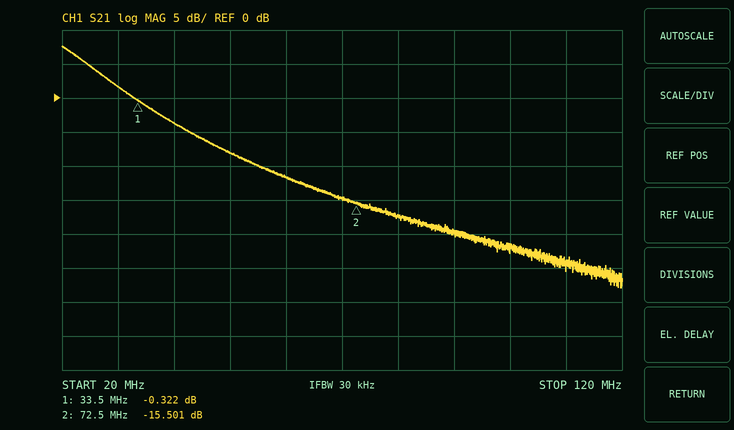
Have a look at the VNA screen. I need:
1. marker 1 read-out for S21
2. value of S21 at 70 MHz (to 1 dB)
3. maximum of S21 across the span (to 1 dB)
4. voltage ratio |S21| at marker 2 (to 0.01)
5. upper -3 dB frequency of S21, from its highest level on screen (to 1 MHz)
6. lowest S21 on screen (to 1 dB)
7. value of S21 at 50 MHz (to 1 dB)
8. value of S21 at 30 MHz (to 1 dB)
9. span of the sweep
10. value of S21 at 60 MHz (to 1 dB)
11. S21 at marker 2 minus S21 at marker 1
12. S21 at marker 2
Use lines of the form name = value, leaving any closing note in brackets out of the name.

marker 1 read-out for S21 = -0.322 dB
value of S21 at 70 MHz = -15 dB
maximum of S21 across the span = 8 dB
voltage ratio |S21| at marker 2 = 0.17
upper -3 dB frequency of S21, from its highest level on screen = 25 MHz
lowest S21 on screen = -28 dB
value of S21 at 50 MHz = -8 dB
value of S21 at 30 MHz = 2 dB
span of the sweep = 100 MHz
value of S21 at 60 MHz = -12 dB
S21 at marker 2 minus S21 at marker 1 = -15.179 dB
S21 at marker 2 = -15.501 dB
